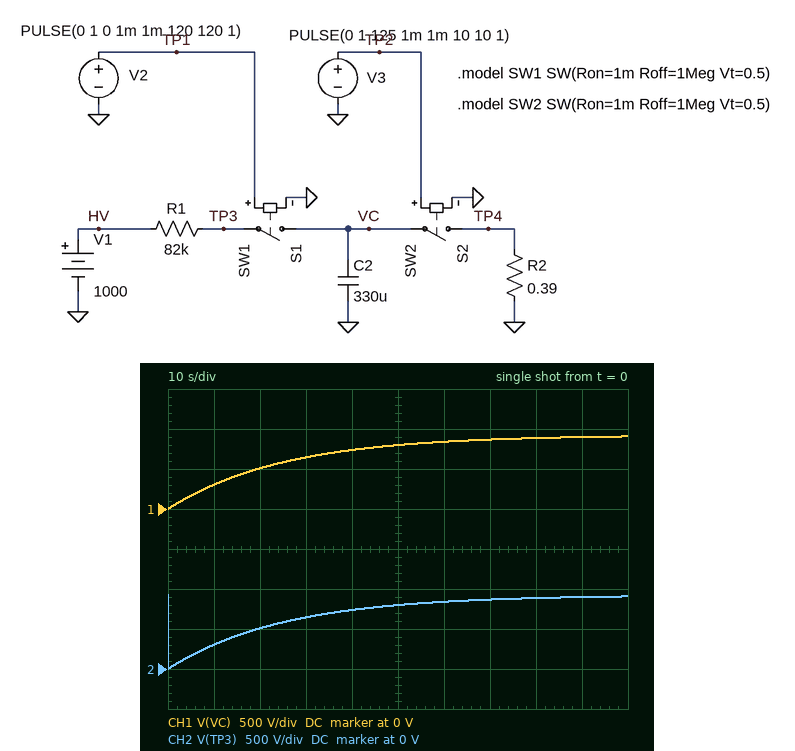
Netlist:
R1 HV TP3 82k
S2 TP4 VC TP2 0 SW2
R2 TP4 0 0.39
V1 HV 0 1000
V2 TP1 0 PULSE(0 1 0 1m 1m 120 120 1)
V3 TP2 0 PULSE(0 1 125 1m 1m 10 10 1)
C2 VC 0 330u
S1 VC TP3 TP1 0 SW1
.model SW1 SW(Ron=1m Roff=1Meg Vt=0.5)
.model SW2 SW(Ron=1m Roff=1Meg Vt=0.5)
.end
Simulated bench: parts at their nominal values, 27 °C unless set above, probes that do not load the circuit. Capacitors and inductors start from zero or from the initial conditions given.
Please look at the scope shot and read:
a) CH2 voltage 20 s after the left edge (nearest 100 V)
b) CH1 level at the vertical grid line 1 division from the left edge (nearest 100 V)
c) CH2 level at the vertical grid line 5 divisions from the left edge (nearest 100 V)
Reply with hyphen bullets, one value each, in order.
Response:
- 500 V
- 300 V
- 800 V
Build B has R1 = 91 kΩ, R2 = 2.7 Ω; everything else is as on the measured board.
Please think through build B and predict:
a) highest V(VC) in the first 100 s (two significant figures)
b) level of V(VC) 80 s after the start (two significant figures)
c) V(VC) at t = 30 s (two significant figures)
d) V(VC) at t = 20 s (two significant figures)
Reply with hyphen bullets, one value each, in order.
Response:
- 890 V
- 870 V
- 610 V
- 470 V
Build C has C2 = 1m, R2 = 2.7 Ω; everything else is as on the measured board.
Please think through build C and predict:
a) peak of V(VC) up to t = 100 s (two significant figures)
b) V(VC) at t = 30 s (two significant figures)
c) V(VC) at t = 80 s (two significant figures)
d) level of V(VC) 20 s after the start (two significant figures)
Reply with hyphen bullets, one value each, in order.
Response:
- 680 V
- 300 V
- 600 V
- 210 V
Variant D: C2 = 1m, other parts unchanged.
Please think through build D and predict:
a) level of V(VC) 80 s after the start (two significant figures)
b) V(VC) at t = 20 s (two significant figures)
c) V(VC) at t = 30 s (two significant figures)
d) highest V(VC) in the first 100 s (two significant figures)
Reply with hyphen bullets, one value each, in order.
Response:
- 600 V
- 210 V
- 300 V
- 680 V
